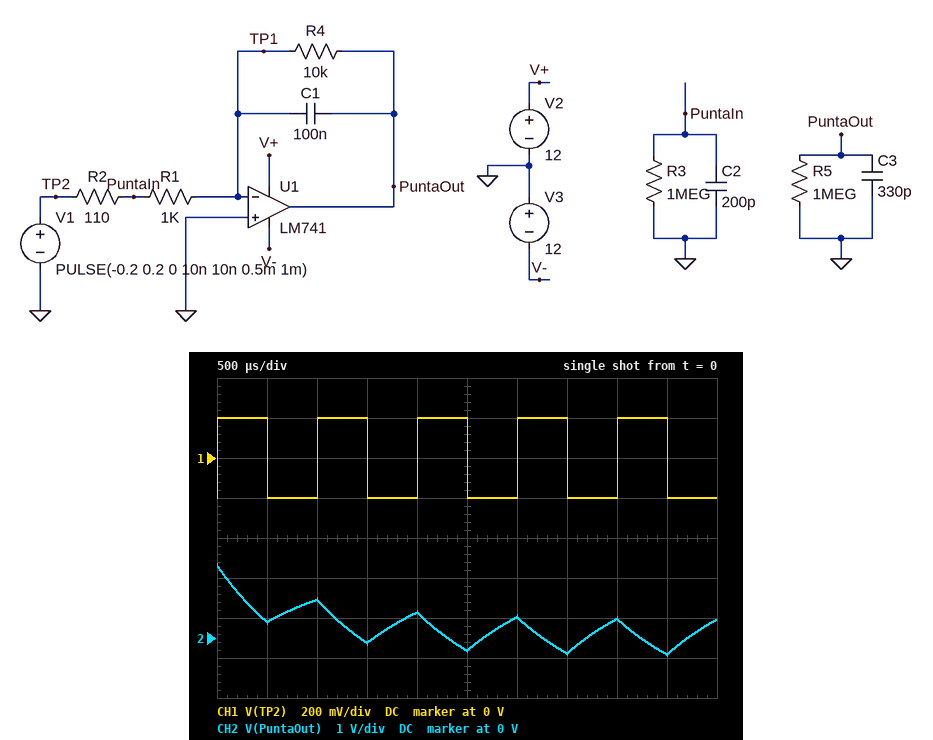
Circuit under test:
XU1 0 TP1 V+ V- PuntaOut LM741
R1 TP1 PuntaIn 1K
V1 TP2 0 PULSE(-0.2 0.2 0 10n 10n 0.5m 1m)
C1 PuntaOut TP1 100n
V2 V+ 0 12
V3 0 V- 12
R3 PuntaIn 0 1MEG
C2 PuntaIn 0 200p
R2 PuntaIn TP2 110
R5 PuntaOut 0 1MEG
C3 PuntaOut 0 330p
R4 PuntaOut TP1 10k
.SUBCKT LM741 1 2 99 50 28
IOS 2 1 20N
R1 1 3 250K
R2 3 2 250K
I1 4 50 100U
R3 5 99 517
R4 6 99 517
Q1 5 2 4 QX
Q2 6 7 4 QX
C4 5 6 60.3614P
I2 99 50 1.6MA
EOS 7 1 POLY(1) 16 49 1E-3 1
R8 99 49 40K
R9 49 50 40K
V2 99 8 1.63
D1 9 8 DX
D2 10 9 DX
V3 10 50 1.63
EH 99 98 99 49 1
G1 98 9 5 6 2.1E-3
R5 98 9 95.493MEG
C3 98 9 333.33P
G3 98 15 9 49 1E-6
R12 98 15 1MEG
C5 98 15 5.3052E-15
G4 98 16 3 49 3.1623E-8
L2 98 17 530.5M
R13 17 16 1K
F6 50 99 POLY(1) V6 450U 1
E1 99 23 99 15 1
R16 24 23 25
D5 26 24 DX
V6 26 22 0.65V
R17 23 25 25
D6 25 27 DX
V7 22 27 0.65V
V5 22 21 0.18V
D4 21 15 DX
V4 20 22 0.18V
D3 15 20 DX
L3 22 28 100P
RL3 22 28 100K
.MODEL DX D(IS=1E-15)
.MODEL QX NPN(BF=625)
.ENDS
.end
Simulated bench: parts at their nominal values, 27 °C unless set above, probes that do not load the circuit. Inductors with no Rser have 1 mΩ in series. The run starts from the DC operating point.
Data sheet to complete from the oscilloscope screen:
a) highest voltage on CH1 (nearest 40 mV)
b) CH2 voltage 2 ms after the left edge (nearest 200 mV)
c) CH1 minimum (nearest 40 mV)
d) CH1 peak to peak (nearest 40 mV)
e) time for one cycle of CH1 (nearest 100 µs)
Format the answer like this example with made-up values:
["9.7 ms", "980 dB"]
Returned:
["200 mV", "600 mV", "-200 mV", "400 mV", "1.0 ms"]
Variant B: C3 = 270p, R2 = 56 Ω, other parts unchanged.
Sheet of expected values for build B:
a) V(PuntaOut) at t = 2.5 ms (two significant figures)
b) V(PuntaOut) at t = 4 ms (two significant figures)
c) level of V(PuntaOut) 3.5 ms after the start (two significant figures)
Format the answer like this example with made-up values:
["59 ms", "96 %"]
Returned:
["-330 mV", "500 mV", "-410 mV"]
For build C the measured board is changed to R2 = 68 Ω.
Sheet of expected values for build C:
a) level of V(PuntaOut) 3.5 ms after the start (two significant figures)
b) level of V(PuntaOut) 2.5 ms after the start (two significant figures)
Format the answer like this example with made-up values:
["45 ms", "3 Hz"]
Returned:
["-400 mV", "-330 mV"]
